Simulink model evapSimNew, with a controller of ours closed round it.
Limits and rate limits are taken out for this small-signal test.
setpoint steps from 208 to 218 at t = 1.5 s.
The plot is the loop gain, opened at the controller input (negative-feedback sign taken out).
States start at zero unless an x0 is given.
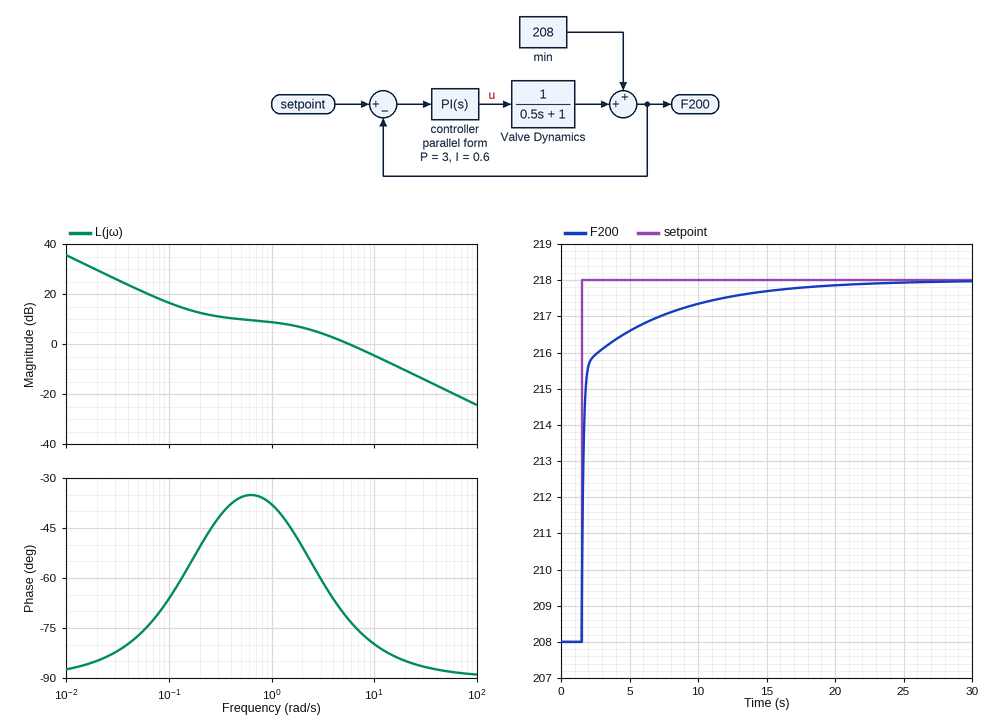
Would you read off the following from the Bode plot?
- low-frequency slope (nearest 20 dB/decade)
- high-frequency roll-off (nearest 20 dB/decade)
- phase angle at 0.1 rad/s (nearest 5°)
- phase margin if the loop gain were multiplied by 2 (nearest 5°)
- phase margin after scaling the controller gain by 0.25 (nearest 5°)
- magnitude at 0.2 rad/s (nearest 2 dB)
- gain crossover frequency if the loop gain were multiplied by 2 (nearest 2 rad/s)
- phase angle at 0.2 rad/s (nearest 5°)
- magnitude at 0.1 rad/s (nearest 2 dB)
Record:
-20 dB/decade
-20 dB/decade
-65°
100°
130°
12 dB
12 rad/s
-50°
16 dB
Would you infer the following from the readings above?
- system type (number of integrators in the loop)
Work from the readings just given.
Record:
1
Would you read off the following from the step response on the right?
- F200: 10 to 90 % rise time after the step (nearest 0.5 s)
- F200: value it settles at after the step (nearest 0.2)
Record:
5.5 s
218.0
